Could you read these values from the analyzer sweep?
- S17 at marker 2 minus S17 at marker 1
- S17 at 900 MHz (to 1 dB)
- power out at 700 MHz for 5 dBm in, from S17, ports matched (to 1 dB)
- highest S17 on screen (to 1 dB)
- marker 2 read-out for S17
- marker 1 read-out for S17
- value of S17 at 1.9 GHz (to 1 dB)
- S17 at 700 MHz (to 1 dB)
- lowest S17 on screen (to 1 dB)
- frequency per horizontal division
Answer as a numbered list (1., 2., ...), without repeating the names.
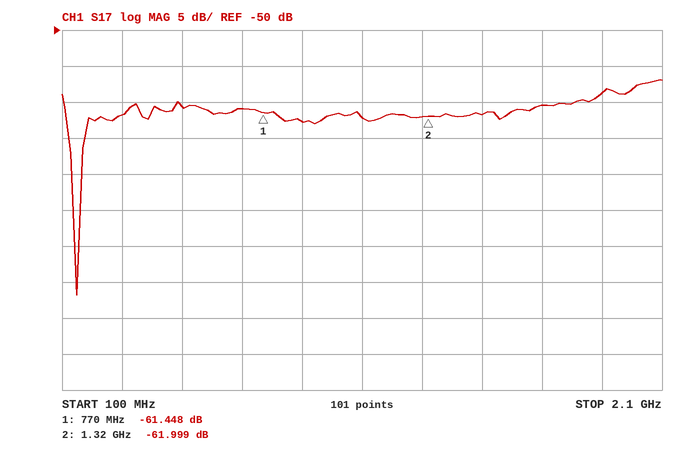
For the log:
1. -0.551 dB
2. -63 dB
3. -56 dBm
4. -57 dB
5. -61.999 dB
6. -61.448 dB
7. -59 dB
8. -61 dB
9. -87 dB
10. 200 MHz
